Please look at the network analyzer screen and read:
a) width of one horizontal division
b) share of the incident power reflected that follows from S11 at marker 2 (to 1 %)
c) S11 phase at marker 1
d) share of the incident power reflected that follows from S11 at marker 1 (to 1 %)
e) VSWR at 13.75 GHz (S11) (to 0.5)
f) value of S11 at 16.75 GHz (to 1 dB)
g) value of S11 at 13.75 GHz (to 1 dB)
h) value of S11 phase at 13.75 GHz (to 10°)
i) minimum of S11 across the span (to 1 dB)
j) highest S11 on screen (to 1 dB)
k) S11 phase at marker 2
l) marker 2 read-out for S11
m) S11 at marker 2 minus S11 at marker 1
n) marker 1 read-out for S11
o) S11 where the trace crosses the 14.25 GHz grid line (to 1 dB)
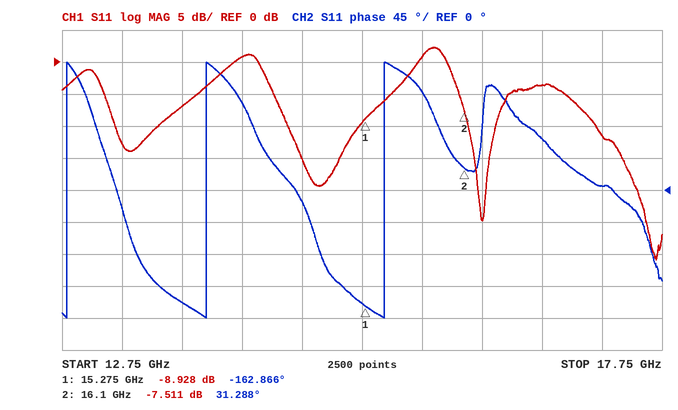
500 MHz
18 %
-162.866°
13 %
2.5
-4 dB
-7 dB
-160°
-31 dB
2 dB
31.288°
-7.511 dB
1.417 dB
-8.928 dB
1 dB
